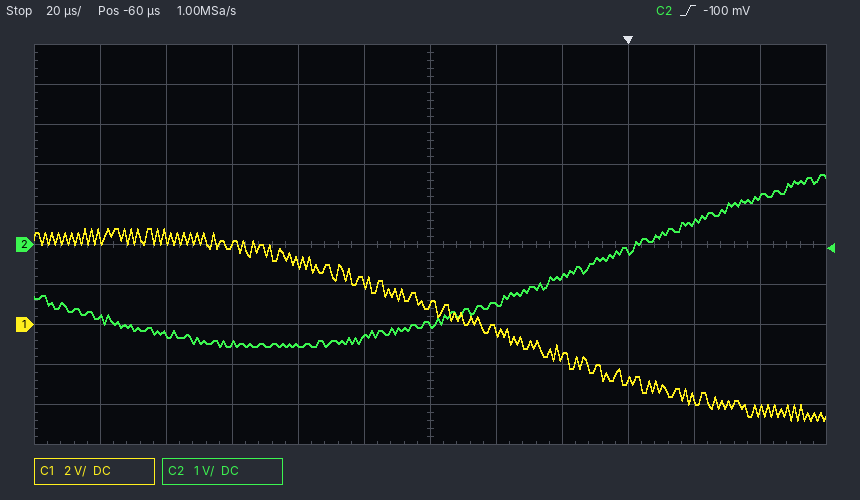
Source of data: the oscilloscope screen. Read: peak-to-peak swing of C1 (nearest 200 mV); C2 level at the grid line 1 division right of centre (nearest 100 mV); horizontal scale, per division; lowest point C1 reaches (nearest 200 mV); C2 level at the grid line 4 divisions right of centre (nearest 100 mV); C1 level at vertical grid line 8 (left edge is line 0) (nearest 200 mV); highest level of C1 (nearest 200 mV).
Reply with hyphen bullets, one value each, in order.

- 9.6 V
- -1.5 V
- 20 µs
- -4.8 V
- 600 mV
- -1.6 V
- 4.8 V
